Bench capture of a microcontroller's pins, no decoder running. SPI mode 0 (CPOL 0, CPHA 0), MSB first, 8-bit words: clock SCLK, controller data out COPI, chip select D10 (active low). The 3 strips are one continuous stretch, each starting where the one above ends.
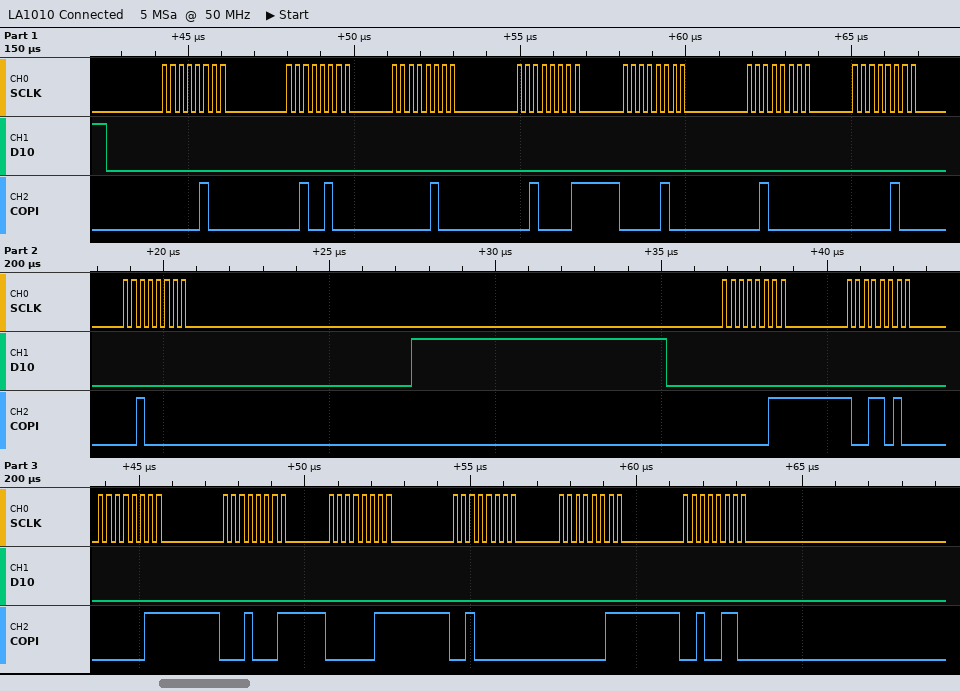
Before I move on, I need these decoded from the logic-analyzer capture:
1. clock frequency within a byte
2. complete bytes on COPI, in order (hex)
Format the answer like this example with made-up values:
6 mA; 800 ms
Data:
4 MHz; 04 24 04 21 04 20 04 20 03 9A 03 11 03 20 03 26
